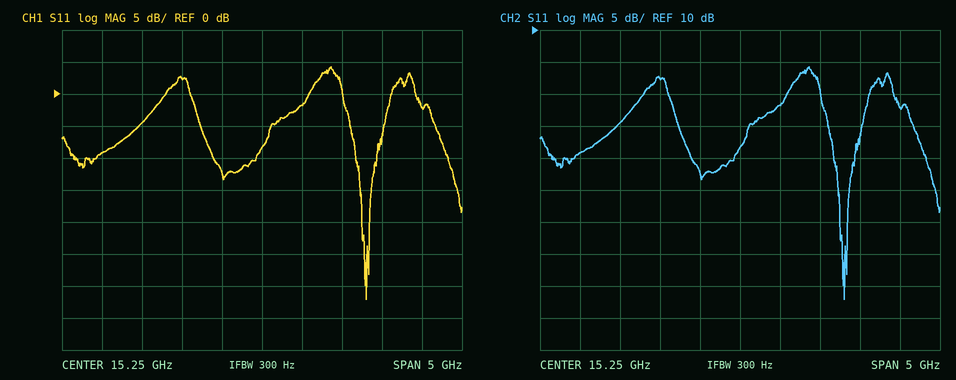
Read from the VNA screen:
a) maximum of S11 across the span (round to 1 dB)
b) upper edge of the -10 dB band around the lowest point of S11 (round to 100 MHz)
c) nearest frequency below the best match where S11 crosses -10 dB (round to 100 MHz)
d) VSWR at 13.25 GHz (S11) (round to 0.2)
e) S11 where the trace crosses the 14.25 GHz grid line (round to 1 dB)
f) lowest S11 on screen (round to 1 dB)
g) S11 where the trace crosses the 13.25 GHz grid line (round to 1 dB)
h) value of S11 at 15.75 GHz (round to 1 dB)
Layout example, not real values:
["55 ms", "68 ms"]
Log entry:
["4 dB", "16.7 GHz", "16.4 GHz", "2.0", "2 dB", "-32 dB", "-9 dB", "-2 dB"]
